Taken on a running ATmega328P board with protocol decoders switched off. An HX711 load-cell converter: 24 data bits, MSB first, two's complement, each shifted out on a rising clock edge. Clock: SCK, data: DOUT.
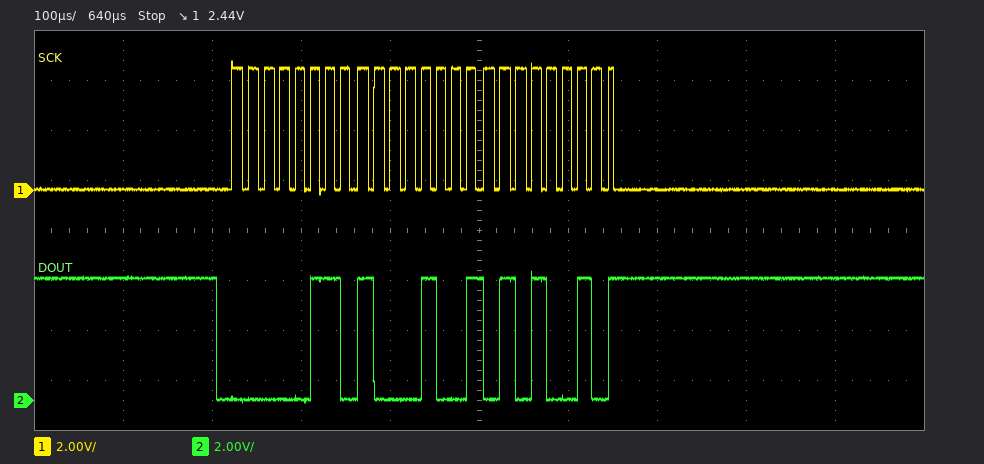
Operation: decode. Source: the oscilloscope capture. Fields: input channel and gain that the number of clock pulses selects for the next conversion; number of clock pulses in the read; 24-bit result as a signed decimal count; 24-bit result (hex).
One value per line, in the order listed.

channel A, gain 128
25
428370
0x068952
